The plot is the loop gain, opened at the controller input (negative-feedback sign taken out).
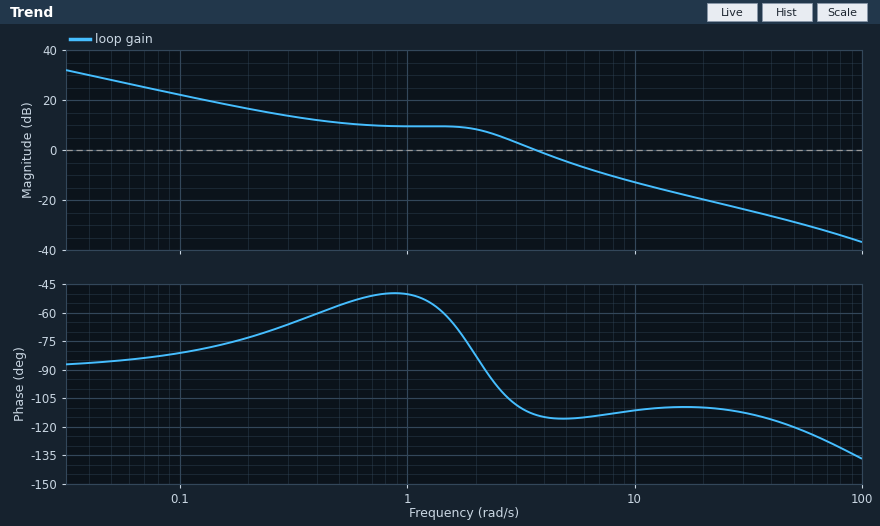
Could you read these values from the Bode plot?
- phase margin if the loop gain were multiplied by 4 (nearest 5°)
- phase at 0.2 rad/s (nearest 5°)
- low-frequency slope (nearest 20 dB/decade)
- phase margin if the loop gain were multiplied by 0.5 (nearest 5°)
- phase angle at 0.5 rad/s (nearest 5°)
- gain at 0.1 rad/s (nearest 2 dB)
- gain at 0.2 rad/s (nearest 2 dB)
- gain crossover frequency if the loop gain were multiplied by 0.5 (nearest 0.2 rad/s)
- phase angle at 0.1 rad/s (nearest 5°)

70°
-75°
-20 dB/decade
80°
-55°
22 dB
16 dB
2.4 rad/s
-80°
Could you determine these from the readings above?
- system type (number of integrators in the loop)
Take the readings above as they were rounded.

1
